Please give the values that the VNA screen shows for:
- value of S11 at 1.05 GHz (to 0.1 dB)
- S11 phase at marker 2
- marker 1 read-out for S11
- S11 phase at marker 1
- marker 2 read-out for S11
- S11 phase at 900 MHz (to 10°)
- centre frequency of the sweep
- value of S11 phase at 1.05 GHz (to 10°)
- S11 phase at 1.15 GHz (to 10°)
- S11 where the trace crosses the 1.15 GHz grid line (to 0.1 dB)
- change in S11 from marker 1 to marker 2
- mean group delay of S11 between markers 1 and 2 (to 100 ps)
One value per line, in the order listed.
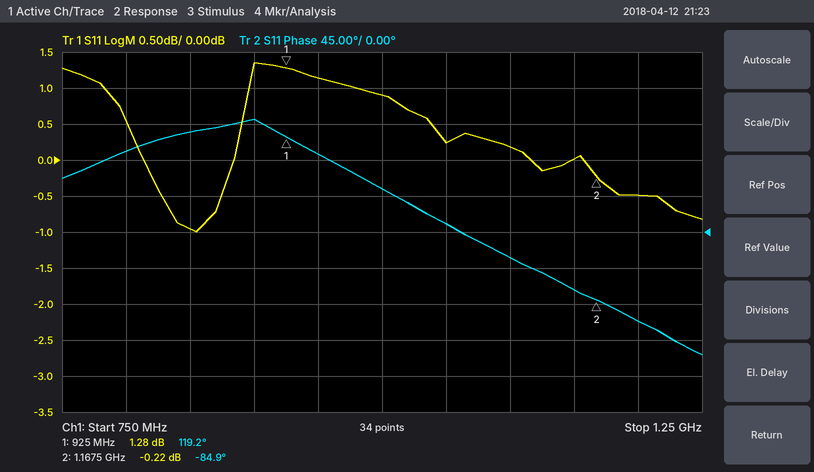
0.2 dB
-84.9°
1.28 dB
119.2°
-0.22 dB
140°
1 GHz
10°
-70°
0.0 dB
-1.50 dB
2.3 ns
